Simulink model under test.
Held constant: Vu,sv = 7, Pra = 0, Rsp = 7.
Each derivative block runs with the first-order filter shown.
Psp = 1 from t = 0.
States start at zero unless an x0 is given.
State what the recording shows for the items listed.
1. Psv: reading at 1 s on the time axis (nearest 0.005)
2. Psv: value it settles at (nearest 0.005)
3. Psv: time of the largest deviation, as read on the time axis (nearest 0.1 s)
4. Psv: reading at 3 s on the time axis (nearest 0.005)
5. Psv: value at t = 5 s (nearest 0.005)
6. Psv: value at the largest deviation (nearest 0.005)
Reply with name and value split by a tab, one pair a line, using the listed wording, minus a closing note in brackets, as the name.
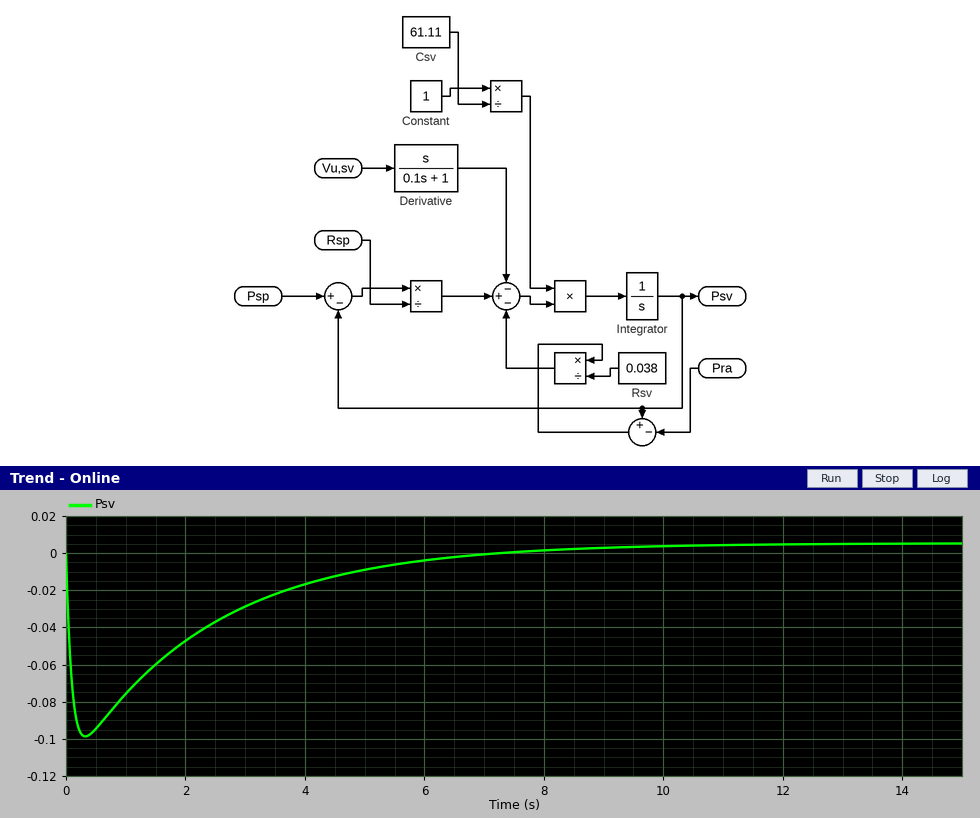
Psv: reading at 1 s on the time axis	-0.075
Psv: value it settles at	0.005
Psv: time of the largest deviation, as read on the time axis	0.3 s
Psv: reading at 3 s on the time axis	-0.030
Psv: value at t = 5 s	-0.010
Psv: value at the largest deviation	-0.100
